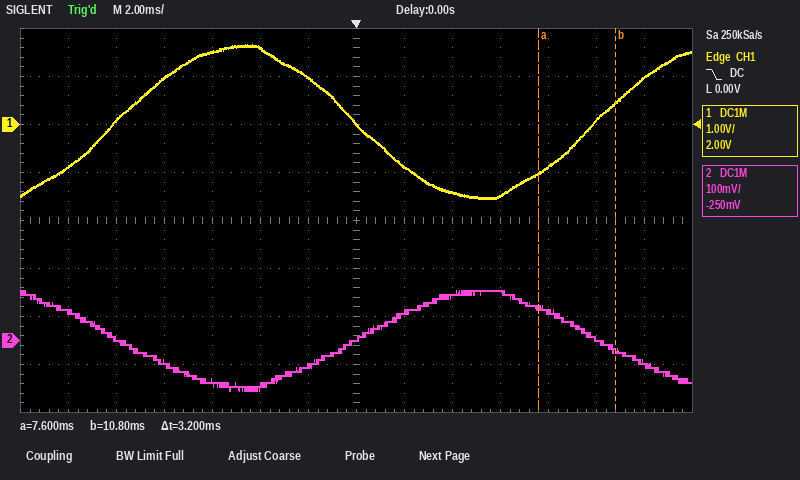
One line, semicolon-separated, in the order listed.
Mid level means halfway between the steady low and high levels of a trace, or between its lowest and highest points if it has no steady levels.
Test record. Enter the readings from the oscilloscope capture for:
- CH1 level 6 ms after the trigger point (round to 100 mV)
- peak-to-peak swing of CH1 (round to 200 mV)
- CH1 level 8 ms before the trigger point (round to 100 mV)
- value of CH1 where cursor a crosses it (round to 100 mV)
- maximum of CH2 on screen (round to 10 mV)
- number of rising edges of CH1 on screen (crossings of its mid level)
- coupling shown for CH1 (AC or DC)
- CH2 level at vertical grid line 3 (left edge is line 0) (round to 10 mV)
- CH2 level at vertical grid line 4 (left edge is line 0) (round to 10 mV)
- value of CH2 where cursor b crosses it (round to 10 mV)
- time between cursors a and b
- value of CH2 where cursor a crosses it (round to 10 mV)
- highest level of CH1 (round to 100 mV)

-1.5 V; 3.2 V; 1.0 V; -1.0 V; 100 mV; 2; DC; -40 mV; -90 mV; -20 mV; 3.2 ms; 70 mV; 1.7 V
